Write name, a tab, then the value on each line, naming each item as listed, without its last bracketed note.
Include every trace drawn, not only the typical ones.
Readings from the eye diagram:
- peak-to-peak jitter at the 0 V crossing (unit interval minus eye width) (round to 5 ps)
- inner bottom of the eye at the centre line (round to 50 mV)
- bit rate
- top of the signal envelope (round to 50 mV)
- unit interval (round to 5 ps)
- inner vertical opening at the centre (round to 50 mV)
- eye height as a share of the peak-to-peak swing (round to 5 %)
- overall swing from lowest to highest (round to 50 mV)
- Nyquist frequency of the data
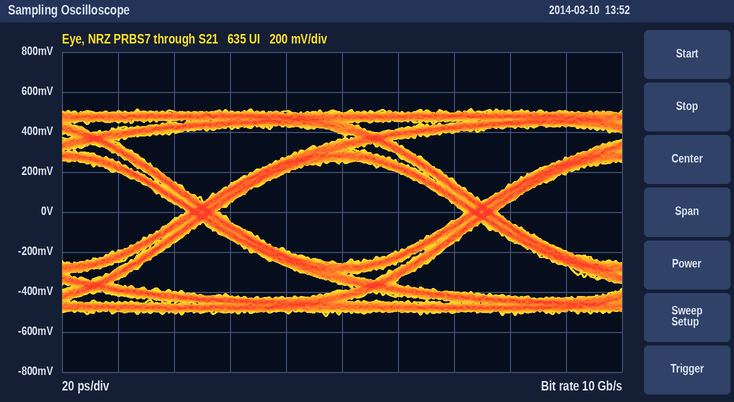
peak-to-peak jitter at the 0 V crossing (unit interval minus eye width)	10 ps
inner bottom of the eye at the centre line	-250 mV
bit rate	10 Gb/s
top of the signal envelope	500 mV
unit interval	100 ps
inner vertical opening at the centre	500 mV
eye height as a share of the peak-to-peak swing	50 %
overall swing from lowest to highest	1.05 V
Nyquist frequency of the data	5 GHz
